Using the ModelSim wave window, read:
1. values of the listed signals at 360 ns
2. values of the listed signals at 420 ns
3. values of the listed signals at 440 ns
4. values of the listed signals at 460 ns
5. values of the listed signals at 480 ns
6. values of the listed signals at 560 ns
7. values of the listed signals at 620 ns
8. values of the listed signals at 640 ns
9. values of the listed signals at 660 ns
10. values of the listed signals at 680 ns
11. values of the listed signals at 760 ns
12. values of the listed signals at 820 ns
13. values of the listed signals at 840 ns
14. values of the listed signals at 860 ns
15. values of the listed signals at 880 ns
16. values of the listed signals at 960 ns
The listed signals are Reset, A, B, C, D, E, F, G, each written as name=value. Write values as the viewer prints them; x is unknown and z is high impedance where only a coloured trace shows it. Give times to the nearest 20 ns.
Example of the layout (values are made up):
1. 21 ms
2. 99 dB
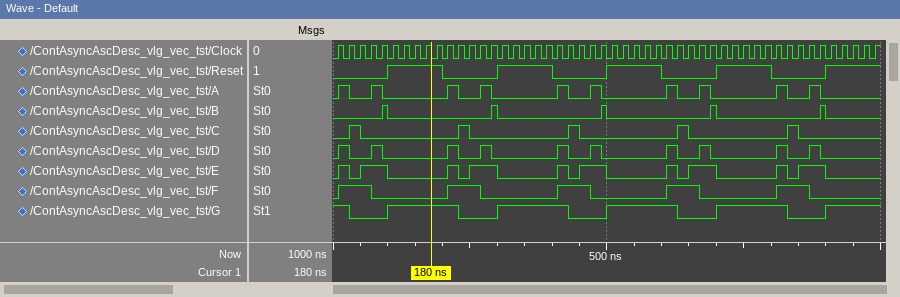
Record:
1. Reset=1, A=0, B=0, C=0, D=0, E=0, F=0, G=1
2. Reset=0, A=1, B=0, C=0, D=1, E=1, F=1, G=1
3. Reset=0, A=0, B=0, C=1, D=0, E=0, F=1, G=0
4. Reset=0, A=0, B=0, C=0, D=0, E=1, F=1, G=0
5. Reset=0, A=1, B=0, C=0, D=1, E=1, F=0, G=0
6. Reset=1, A=0, B=0, C=0, D=0, E=0, F=0, G=1
7. Reset=0, A=1, B=0, C=0, D=1, E=1, F=1, G=1
8. Reset=0, A=0, B=0, C=1, D=0, E=0, F=1, G=0
9. Reset=0, A=0, B=0, C=0, D=0, E=1, F=1, G=0
10. Reset=0, A=1, B=0, C=0, D=1, E=1, F=0, G=0
11. Reset=1, A=0, B=0, C=0, D=0, E=0, F=0, G=1
12. Reset=0, A=1, B=0, C=0, D=1, E=1, F=1, G=1
13. Reset=0, A=0, B=0, C=1, D=0, E=0, F=1, G=0
14. Reset=0, A=0, B=0, C=0, D=0, E=1, F=1, G=0
15. Reset=0, A=1, B=0, C=0, D=1, E=1, F=0, G=0
16. Reset=1, A=0, B=0, C=0, D=0, E=0, F=0, G=1
